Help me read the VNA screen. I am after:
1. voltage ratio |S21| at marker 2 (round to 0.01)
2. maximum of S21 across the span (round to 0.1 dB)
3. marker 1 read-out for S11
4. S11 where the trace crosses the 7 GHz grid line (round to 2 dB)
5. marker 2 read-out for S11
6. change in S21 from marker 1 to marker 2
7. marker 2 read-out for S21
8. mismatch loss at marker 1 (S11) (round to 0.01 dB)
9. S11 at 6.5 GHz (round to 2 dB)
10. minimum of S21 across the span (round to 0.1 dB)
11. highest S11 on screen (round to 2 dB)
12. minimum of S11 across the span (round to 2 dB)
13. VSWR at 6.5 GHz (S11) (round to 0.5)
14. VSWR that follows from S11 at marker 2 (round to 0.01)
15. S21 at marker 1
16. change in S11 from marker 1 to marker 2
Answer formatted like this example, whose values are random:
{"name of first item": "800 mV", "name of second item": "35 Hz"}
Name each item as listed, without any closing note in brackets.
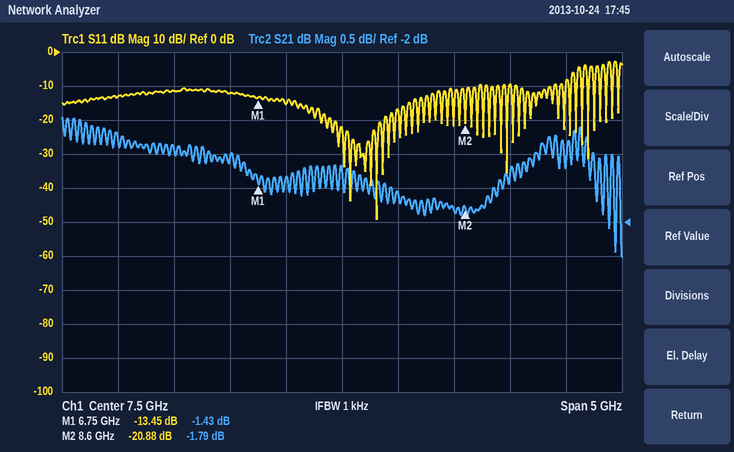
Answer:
{"voltage ratio |S21| at marker 2": "0.81", "maximum of S21 across the span": "-0.5 dB", "marker 1 read-out for S11": "-13.45 dB", "S11 where the trace crosses the 7 GHz grid line": "-16 dB", "marker 2 read-out for S11": "-20.88 dB", "change in S21 from marker 1 to marker 2": "-0.36 dB", "marker 2 read-out for S21": "-1.79 dB", "mismatch loss at marker 1 (S11)": "0.20 dB", "S11 at 6.5 GHz": "-12 dB", "minimum of S21 across the span": "-2.5 dB", "highest S11 on screen": "-2 dB", "minimum of S11 across the span": "-50 dB", "VSWR at 6.5 GHz (S11)": "1.5", "VSWR that follows from S11 at marker 2": "1.20", "S21 at marker 1": "-1.43 dB", "change in S11 from marker 1 to marker 2": "-7.43 dB"}
